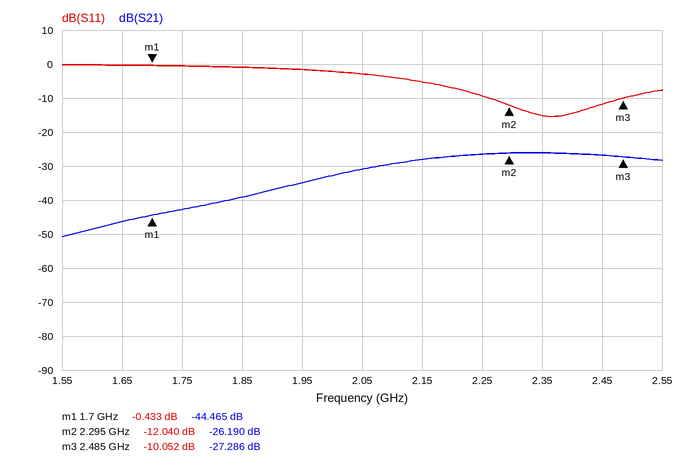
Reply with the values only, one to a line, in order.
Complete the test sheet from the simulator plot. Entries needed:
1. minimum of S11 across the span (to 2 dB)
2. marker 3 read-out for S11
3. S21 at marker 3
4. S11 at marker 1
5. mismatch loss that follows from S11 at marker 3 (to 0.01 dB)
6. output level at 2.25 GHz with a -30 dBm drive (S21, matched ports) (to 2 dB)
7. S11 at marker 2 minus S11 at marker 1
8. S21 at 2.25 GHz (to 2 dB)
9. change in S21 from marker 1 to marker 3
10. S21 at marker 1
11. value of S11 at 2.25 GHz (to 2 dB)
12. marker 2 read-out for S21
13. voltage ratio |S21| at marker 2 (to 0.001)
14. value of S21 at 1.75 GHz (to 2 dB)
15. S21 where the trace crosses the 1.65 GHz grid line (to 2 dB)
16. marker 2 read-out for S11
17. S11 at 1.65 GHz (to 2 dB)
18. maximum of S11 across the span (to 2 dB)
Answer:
-16 dB
-10.052 dB
-27.286 dB
-0.433 dB
0.45 dB
-56 dBm
-11.607 dB
-26 dB
17.179 dB
-44.465 dB
-10 dB
-26.190 dB
0.049
-42 dB
-46 dB
-12.040 dB
0 dB
0 dB
